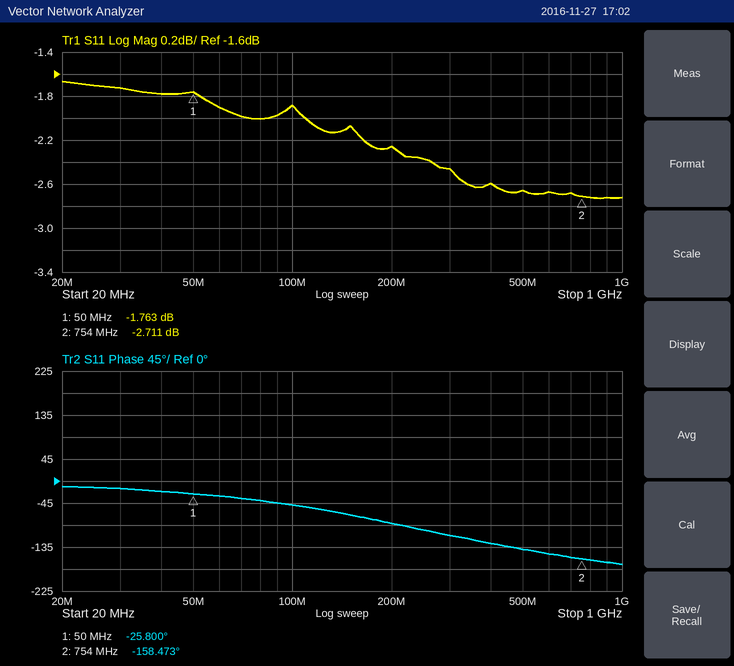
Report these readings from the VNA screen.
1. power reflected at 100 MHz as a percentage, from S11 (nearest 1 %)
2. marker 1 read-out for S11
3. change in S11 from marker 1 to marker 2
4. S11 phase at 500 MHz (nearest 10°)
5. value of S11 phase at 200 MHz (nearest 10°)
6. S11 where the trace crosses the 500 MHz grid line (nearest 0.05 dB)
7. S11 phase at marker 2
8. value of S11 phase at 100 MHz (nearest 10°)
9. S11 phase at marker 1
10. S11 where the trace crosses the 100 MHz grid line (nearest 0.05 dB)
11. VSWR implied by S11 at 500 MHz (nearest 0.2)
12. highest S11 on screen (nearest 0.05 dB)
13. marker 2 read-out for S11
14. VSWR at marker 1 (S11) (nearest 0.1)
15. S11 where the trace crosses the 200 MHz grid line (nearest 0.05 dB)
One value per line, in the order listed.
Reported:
65 %
-1.763 dB
-0.948 dB
-140°
-90°
-2.65 dB
-158.473°
-50°
-25.800°
-1.90 dB
6.6
-1.65 dB
-2.711 dB
9.9
-2.25 dB
